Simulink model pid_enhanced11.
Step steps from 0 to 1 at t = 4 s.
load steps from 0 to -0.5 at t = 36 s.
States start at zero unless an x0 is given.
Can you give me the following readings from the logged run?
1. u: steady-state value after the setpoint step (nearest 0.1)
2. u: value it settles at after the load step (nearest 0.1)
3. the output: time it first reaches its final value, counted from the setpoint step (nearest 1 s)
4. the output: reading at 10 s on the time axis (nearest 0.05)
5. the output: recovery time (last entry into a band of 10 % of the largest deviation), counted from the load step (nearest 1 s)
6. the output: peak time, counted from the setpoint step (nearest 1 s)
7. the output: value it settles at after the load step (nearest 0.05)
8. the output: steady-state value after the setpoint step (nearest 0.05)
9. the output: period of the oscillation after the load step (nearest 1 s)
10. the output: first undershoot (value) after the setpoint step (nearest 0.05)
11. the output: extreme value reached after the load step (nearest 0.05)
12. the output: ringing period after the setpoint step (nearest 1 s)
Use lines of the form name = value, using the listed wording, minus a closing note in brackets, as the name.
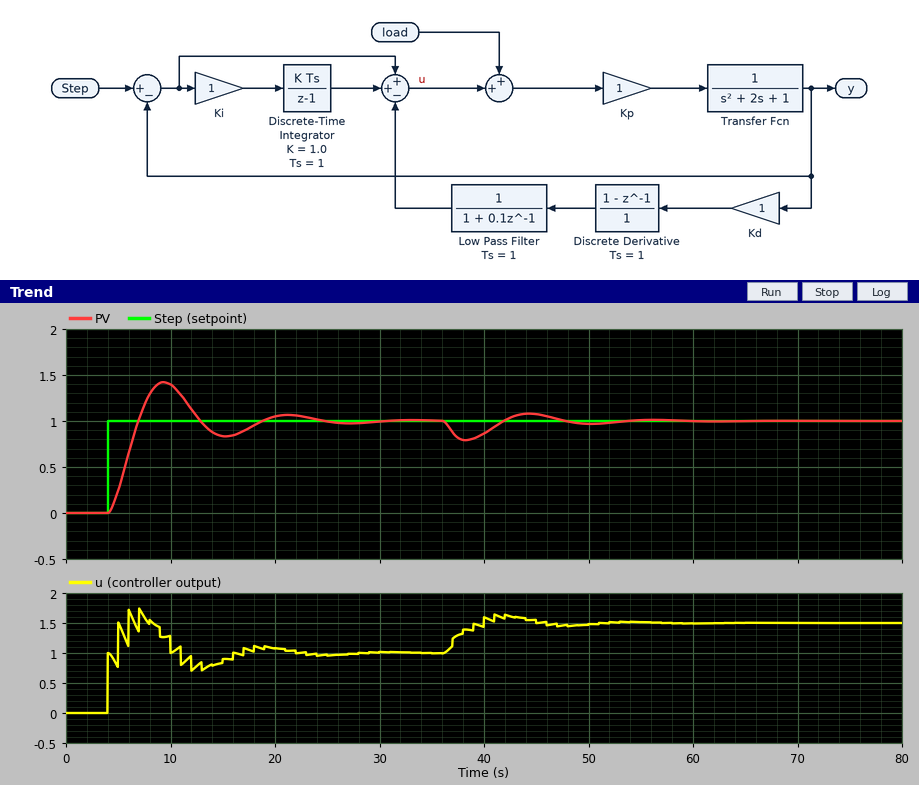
u: steady-state value after the setpoint step = 1.0
u: value it settles at after the load step = 1.5
the output: time it first reaches its final value, counted from the setpoint step = 3 s
the output: reading at 10 s on the time axis = 1.40
the output: recovery time (last entry into a band of 10 % of the largest deviation), counted from the load step = 16 s
the output: peak time, counted from the setpoint step = 5 s
the output: value it settles at after the load step = 1.00
the output: steady-state value after the setpoint step = 1.00
the output: period of the oscillation after the load step = 12 s
the output: first undershoot (value) after the setpoint step = 0.85
the output: extreme value reached after the load step = 0.80
the output: ringing period after the setpoint step = 12 s
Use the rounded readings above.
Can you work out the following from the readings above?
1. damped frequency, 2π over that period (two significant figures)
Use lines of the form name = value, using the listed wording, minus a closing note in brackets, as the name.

damped frequency, 2π over that period = 0.52 rad/s
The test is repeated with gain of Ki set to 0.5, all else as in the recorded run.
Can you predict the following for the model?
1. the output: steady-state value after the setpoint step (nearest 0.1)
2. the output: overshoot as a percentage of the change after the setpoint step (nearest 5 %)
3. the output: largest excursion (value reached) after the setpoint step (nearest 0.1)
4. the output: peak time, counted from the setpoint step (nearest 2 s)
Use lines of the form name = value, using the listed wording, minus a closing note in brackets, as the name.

the output: steady-state value after the setpoint step = 1.0
the output: overshoot as a percentage of the change after the setpoint step = 10 %
the output: largest excursion (value reached) after the setpoint step = 1.1
the output: peak time, counted from the setpoint step = 8 s
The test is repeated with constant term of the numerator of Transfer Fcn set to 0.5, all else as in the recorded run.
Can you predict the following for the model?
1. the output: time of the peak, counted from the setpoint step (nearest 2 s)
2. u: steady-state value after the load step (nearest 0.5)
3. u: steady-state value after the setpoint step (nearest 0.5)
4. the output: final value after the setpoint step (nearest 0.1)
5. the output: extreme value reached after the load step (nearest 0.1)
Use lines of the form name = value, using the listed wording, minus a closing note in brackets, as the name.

the output: time of the peak, counted from the setpoint step = 8 s
u: steady-state value after the load step = 2.5
u: steady-state value after the setpoint step = 2.0
the output: final value after the setpoint step = 1.0
the output: extreme value reached after the load step = 0.9
